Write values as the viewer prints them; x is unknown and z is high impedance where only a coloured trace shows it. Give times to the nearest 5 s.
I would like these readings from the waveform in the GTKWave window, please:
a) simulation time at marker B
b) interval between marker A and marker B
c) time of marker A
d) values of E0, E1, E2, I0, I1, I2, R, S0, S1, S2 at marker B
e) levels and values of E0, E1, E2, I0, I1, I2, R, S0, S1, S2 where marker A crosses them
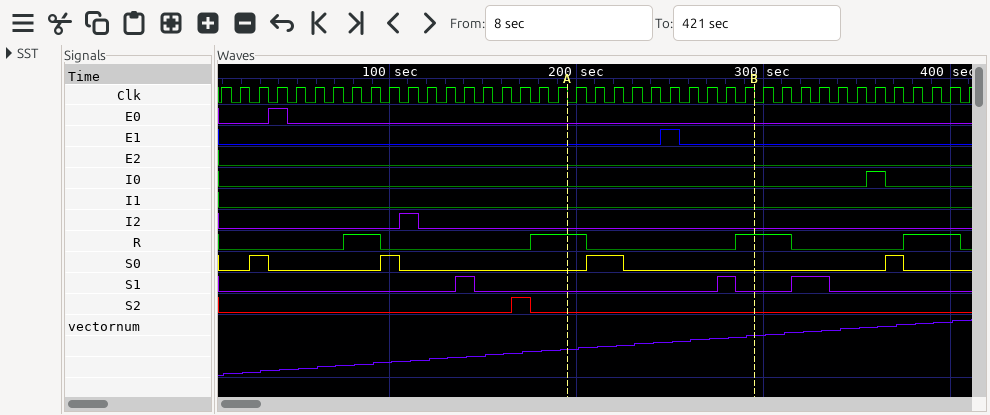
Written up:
295 s
100 s
195 s
E0=0, E1=0, E2=0, I0=0, I1=0, I2=0, R=1, S0=0, S1=0, S2=0
E0=0, E1=0, E2=0, I0=0, I1=0, I2=0, R=1, S0=0, S1=0, S2=0
